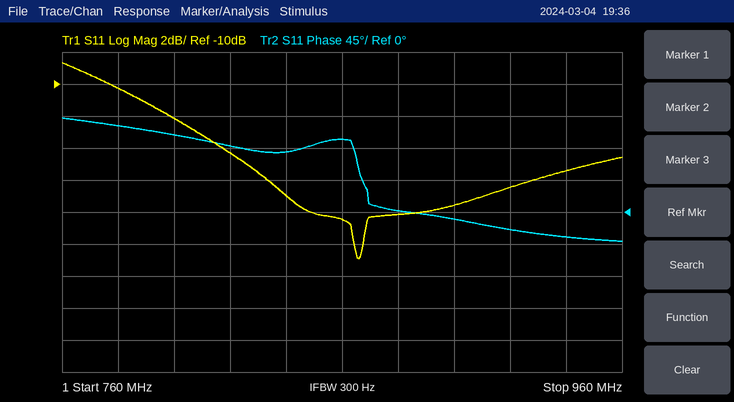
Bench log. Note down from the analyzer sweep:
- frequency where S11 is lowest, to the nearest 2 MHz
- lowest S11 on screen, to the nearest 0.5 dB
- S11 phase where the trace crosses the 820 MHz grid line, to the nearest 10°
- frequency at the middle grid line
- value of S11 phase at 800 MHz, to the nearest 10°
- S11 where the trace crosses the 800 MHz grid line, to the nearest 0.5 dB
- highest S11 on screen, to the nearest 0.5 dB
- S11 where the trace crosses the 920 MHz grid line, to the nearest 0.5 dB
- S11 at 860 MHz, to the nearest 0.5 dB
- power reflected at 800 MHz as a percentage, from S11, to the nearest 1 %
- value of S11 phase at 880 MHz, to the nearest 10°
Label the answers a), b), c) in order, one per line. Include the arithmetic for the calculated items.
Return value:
a) 866 MHz
b) -21.0 dB
c) 90°
d) 860 MHz
e) 110°
f) -12.0 dB
g) -8.5 dB
h) -16.5 dB
i) -18.5 dB
j) 10^(-12/10) ≈ 6 %
k) 0°
